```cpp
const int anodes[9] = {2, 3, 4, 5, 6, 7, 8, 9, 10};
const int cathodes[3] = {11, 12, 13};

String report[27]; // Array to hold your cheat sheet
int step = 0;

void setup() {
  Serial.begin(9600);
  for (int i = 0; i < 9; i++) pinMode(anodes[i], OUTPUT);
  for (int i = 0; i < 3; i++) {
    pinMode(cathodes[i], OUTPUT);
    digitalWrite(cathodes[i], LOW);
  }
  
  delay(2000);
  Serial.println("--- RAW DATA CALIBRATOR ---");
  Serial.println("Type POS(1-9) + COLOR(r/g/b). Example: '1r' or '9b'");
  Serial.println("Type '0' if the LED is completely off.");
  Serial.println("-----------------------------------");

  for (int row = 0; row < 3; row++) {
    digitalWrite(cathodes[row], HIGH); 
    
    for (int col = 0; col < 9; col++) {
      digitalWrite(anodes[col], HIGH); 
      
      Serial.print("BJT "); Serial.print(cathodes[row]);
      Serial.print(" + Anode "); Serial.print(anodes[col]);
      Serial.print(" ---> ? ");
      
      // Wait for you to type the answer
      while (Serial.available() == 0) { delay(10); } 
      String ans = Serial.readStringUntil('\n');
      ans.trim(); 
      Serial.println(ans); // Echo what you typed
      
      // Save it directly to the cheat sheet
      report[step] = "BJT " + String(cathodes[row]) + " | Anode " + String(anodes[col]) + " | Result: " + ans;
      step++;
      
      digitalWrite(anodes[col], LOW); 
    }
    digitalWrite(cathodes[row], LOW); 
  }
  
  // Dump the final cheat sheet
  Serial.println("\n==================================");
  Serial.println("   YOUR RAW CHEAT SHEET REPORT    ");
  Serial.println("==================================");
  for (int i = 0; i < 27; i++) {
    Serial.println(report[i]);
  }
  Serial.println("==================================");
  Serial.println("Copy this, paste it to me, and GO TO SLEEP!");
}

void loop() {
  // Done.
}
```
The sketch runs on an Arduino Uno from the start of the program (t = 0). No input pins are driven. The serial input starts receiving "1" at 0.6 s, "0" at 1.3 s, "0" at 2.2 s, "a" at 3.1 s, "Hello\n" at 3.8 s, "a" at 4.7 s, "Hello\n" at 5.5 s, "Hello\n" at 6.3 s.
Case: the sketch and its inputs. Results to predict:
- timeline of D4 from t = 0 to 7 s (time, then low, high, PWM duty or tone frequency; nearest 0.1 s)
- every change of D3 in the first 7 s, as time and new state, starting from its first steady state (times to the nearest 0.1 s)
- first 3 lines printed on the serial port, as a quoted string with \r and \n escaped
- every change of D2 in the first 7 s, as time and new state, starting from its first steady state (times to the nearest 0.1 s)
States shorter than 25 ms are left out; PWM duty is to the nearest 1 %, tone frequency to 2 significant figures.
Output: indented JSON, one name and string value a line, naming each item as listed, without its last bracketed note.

{
  "timeline of D4 from t = 0 to 7 s": "0 s low; 5.5 s high; 6.3 s low",
  "every change of D3 in the first 7 s, as time and new state, starting from its first steady state": "0 s low; 3.8 s high; 5.5 s low",
  "first 3 lines printed on the serial port, as a quoted string with \\r and \\n escaped": "\"--- RAW DATA CALIBRATOR ---\\r\\nType POS(1-9) + COLOR(r/g/b). Example: '1r' or '9b'\\r\\nType '0' if the LED is completely off.\\r\\n\"",
  "every change of D2 in the first 7 s, as time and new state, starting from its first steady state": "0 s low; 2.1 s high; 3.8 s low"
}
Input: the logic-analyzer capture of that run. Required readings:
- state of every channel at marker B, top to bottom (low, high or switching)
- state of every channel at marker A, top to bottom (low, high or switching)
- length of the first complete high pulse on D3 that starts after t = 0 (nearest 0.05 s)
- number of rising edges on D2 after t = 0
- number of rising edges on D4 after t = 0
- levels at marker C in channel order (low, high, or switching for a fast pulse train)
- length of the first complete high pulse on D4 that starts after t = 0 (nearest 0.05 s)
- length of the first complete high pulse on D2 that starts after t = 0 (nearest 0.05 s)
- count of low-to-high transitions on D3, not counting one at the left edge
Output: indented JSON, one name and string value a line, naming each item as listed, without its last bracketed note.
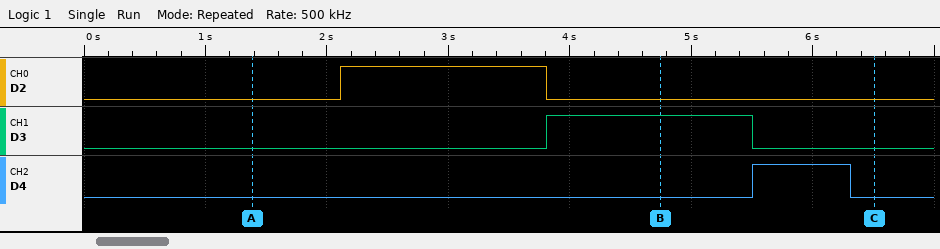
{
  "state of every channel at marker B, top to bottom": "D2 low, D3 high, D4 low",
  "state of every channel at marker A, top to bottom": "D2 low, D3 low, D4 low",
  "length of the first complete high pulse on D3 that starts after t = 0": "1.70 s",
  "number of rising edges on D2 after t = 0": "1",
  "number of rising edges on D4 after t = 0": "1",
  "levels at marker C in channel order": "D2 low, D3 low, D4 low",
  "length of the first complete high pulse on D4 that starts after t = 0": "0.80 s",
  "length of the first complete high pulse on D2 that starts after t = 0": "1.70 s",
  "count of low-to-high transitions on D3, not counting one at the left edge": "1"
}
